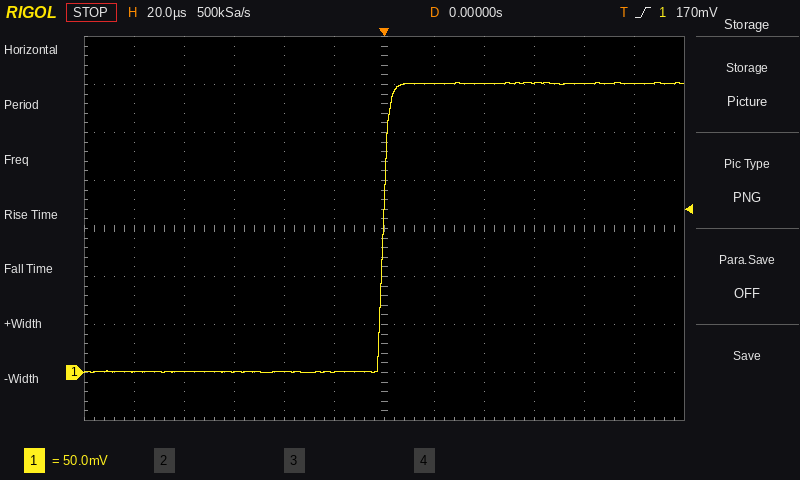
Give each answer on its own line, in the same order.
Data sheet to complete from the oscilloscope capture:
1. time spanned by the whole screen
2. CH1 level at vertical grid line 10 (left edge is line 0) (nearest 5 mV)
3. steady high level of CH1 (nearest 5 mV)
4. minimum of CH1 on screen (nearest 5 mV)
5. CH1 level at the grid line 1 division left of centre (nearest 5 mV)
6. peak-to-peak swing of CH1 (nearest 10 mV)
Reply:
240 µs
300 mV
300 mV
0 mV
0 mV
300 mV
